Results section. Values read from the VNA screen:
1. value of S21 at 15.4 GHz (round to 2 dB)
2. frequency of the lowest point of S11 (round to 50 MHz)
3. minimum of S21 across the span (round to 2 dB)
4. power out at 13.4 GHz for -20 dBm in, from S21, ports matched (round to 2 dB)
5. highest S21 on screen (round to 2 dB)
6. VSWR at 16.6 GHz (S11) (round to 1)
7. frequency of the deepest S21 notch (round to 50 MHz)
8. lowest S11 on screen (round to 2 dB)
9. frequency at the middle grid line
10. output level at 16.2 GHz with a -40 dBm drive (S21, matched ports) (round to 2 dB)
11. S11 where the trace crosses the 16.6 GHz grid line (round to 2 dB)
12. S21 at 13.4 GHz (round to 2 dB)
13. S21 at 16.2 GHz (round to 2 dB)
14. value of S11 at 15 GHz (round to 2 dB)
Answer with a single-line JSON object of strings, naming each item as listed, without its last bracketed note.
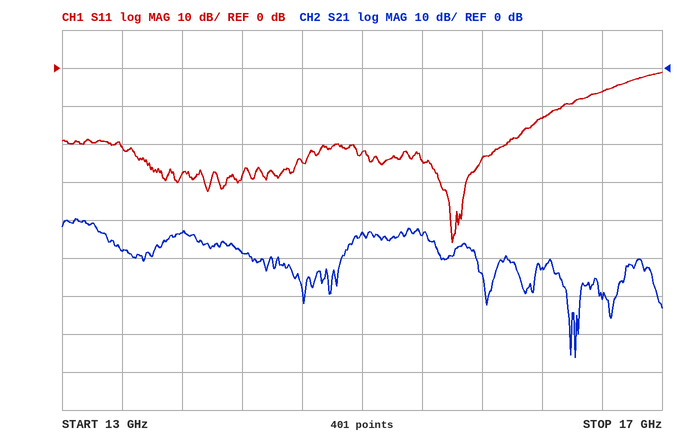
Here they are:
{"value of S21 at 15.4 GHz": "-44 dB", "frequency of the lowest point of S11": "15.60 GHz", "minimum of S21 across the span": "-76 dB", "power out at 13.4 GHz for -20 dBm in, from S21, ports matched": "-68 dBm", "highest S21 on screen": "-40 dB", "VSWR at 16.6 GHz (S11)": "3", "frequency of the deepest S21 notch": "16.40 GHz", "lowest S11 on screen": "-46 dB", "frequency at the middle grid line": "15 GHz", "output level at 16.2 GHz with a -40 dBm drive (S21, matched ports)": "-92 dBm", "S11 where the trace crosses the 16.6 GHz grid line": "-6 dB", "S21 at 13.4 GHz": "-48 dB", "S21 at 16.2 GHz": "-52 dB", "value of S11 at 15 GHz": "-22 dB"}
